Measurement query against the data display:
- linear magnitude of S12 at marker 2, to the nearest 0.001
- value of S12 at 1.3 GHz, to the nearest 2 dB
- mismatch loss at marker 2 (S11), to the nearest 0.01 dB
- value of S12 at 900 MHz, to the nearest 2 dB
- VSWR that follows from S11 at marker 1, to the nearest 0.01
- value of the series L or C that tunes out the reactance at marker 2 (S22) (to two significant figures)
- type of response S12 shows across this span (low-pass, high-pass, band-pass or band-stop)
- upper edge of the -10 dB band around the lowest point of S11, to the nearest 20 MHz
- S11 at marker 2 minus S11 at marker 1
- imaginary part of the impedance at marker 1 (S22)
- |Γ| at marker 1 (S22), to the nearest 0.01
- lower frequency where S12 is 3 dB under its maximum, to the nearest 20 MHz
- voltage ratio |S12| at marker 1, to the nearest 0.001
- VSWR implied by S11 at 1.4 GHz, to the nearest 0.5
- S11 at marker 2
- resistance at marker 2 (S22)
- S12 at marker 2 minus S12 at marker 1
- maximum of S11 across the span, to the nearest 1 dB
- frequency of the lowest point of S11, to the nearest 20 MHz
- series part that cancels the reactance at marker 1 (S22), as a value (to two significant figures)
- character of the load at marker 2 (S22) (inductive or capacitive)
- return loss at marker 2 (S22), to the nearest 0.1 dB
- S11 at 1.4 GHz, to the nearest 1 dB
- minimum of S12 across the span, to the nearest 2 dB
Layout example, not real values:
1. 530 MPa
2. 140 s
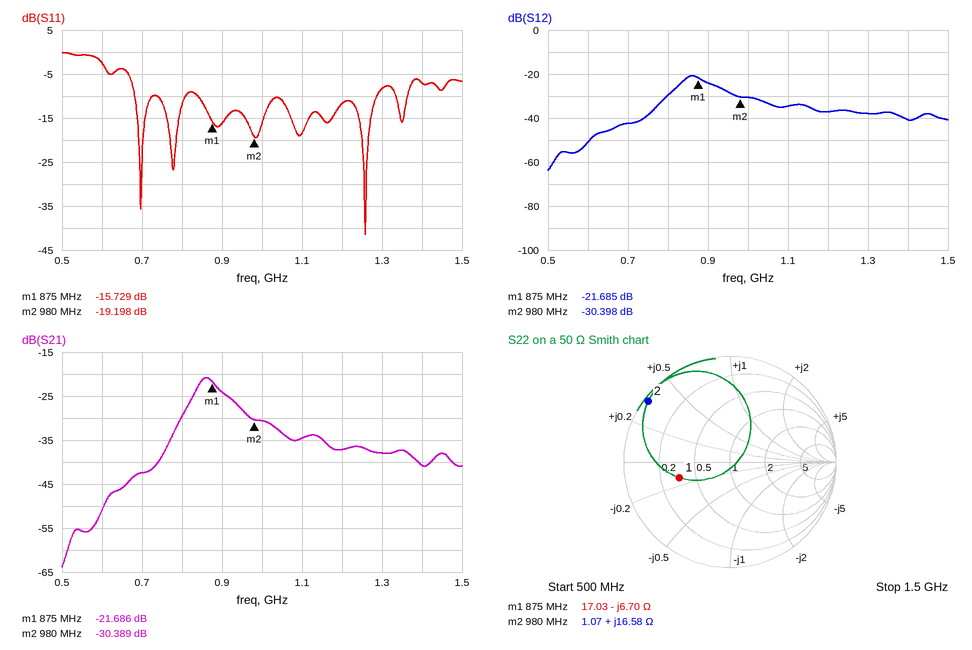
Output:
1. 0.030
2. -38 dB
3. 0.05 dB
4. -24 dB
5. 1.39
6. 9.8 pF
7. band-pass
8. 1.28 GHz
9. -3.469 dB
10. -6.70 Ω
11. 0.50
12. 840 MHz
13. 0.082
14. 2.5
15. -19.198 dB
16. 1.07 Ω
17. -8.713 dB
18. 0 dB
19. 1.26 GHz
20. 1.2 nH
21. inductive
22. 0.3 dB
23. -7 dB
24. -64 dB
